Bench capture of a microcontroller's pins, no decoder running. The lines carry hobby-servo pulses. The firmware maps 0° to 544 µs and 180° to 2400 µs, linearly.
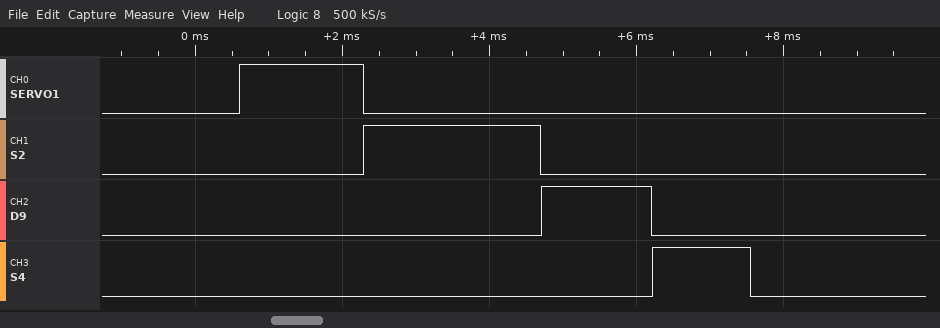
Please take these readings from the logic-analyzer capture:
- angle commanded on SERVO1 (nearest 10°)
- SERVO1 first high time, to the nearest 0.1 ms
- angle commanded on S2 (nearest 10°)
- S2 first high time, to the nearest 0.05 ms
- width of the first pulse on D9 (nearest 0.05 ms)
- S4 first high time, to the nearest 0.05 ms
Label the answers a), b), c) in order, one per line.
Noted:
a) 110°
b) 1.7 ms
c) 180°
d) 2.40 ms
e) 1.50 ms
f) 1.35 ms
